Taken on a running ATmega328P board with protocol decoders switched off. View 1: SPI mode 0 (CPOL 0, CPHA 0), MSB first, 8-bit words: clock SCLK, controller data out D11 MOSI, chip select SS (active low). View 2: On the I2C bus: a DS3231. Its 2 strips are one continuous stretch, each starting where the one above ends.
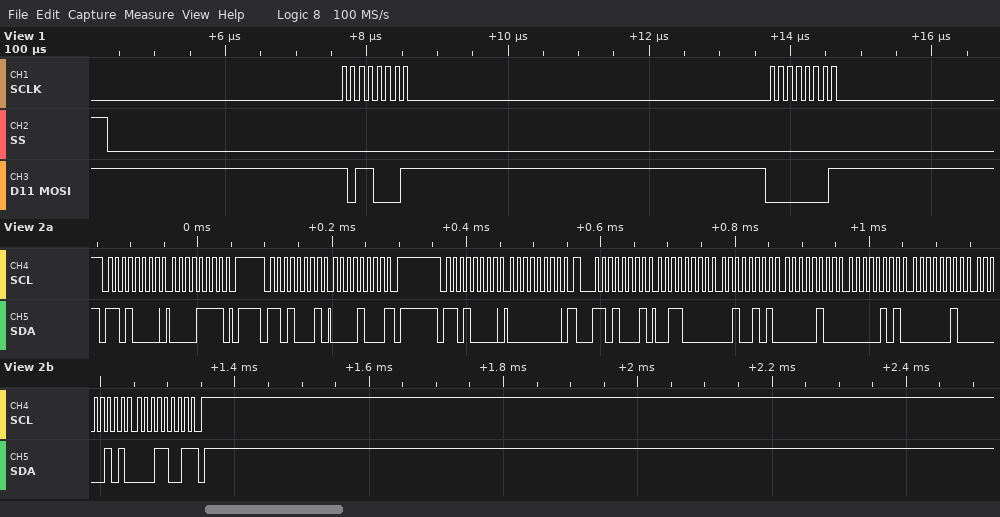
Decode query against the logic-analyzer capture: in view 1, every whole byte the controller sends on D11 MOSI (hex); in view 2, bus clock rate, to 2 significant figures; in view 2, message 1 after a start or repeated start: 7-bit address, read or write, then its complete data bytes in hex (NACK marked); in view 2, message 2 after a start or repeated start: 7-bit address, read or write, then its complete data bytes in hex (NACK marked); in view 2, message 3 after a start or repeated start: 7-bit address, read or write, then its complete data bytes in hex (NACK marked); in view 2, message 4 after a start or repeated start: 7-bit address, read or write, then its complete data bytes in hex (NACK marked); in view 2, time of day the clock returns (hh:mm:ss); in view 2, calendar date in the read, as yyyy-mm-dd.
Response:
B1 01
100 kHz
0x68 write: 0F
0x68 read: 08 NACK
0x68 write: 00
0x68 read: 30 25 04 05 02 05 19 NACK
04:25:30
2019-05-02
